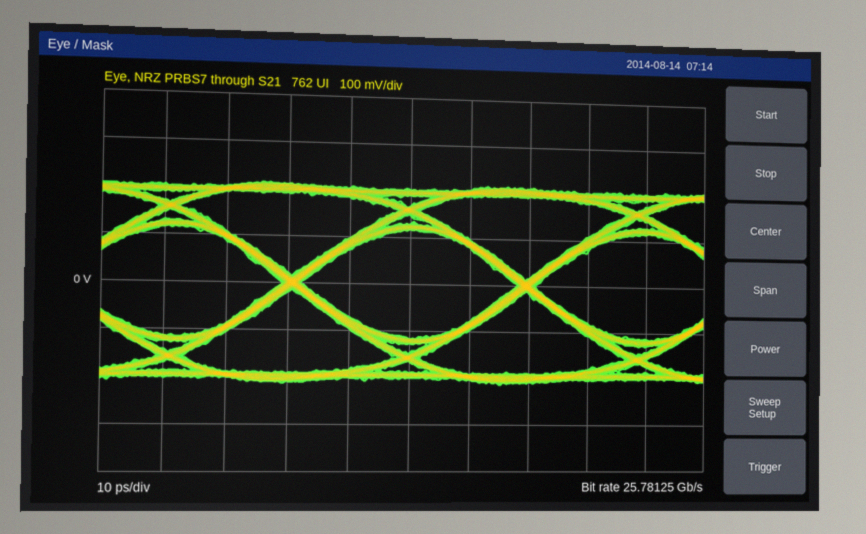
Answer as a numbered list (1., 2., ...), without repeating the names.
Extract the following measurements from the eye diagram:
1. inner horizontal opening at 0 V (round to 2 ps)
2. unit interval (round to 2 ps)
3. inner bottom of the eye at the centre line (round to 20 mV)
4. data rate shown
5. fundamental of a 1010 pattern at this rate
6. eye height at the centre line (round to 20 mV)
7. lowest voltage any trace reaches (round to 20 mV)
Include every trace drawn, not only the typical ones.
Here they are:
1. 36 ps
2. 38 ps
3. -120 mV
4. 25.78125 Gb/s
5. 12.89062 GHz
6. 240 mV
7. -220 mV
